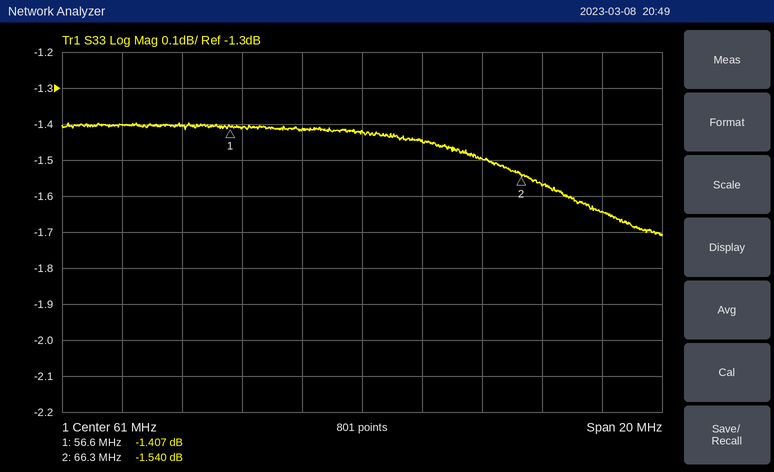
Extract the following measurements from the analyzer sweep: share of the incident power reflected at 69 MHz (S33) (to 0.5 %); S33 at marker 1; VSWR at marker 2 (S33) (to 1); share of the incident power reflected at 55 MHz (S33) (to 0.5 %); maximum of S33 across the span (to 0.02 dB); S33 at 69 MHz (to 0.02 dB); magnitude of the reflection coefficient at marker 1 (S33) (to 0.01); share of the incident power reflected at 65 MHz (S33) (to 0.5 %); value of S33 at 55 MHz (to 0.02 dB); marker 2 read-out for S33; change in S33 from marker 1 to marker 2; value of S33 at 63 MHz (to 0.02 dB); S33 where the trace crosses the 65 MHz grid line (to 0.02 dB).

68.5 %
-1.407 dB
11
72.5 %
-1.40 dB
-1.64 dB
0.85
71.0 %
-1.40 dB
-1.540 dB
-0.133 dB
-1.44 dB
-1.50 dB
